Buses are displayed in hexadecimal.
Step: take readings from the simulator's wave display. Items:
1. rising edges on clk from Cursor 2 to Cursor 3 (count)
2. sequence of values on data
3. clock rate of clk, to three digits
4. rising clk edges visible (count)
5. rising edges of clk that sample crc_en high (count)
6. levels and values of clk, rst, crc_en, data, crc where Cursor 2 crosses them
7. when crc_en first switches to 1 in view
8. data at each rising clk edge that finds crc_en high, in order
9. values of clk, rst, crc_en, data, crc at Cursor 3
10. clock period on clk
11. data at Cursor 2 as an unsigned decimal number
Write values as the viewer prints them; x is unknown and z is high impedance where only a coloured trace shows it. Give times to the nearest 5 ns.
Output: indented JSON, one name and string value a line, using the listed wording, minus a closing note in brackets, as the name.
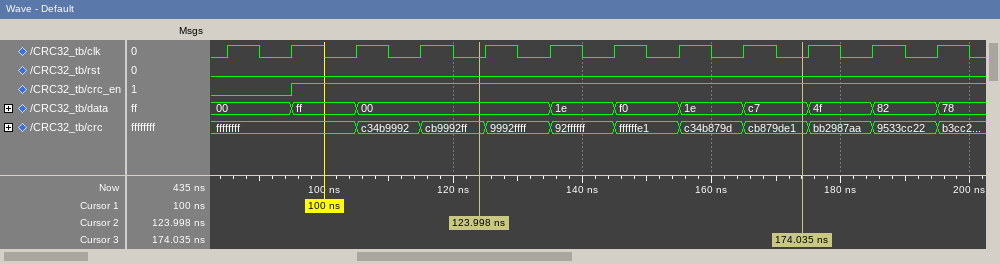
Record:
{
  "rising edges on clk from Cursor 2 to Cursor 3": "5",
  "sequence of values on data": "00, ff, 00, 1e, f0, 1e, c7, 4f, 82, 78",
  "clock rate of clk, to three digits": "100 MHz",
  "rising clk edges visible": "12",
  "rising edges of clk that sample crc_en high": "10",
  "levels and values of clk, rst, crc_en, data, crc where Cursor 2 crosses them": "clk=0, rst=0, crc_en=1, data=00, crc=cb9992ff",
  "when crc_en first switches to 1 in view": "95 ns",
  "data at each rising clk edge that finds crc_en high, in order": "ff, 00, 00, 00, 1e, f0, 1e, c7, 4f, 82",
  "values of clk, rst, crc_en, data, crc at Cursor 3": "clk=0, rst=0, crc_en=1, data=c7, crc=cb879de1",
  "clock period on clk": "10 ns",
  "data at Cursor 2 as an unsigned decimal number": "0"
}
